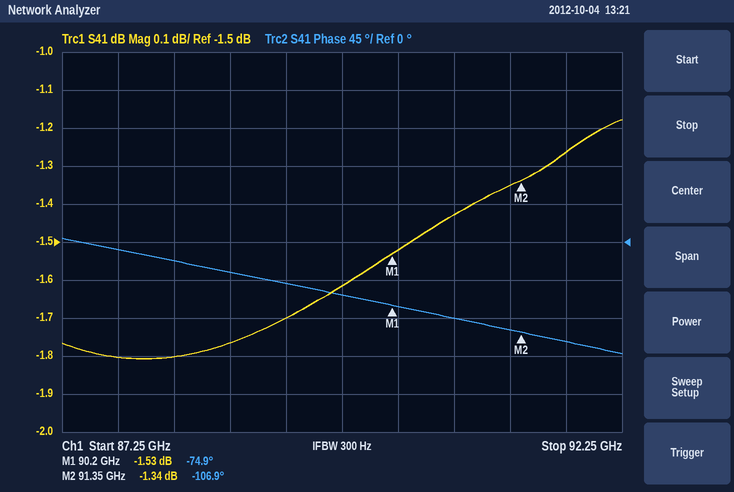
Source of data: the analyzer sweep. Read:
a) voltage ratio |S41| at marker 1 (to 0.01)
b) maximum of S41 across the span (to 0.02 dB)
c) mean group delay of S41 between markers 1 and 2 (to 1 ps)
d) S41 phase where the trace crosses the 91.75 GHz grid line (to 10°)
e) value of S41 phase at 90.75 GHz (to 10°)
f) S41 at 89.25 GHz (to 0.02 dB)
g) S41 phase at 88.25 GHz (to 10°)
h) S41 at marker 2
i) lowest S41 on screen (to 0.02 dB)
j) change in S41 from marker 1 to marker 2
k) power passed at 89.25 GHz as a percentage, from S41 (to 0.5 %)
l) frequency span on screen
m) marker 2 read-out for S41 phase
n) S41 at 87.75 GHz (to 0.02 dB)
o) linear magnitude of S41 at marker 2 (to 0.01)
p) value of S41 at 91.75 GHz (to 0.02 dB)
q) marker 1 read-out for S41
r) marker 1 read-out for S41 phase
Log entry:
0.84
-1.18 dB
77 ps
-120°
-90°
-1.70 dB
-20°
-1.34 dB
-1.80 dB
0.19 dB
67.5 %
5 GHz
-106.9°
-1.80 dB
0.86
-1.26 dB
-1.53 dB
-74.9°
